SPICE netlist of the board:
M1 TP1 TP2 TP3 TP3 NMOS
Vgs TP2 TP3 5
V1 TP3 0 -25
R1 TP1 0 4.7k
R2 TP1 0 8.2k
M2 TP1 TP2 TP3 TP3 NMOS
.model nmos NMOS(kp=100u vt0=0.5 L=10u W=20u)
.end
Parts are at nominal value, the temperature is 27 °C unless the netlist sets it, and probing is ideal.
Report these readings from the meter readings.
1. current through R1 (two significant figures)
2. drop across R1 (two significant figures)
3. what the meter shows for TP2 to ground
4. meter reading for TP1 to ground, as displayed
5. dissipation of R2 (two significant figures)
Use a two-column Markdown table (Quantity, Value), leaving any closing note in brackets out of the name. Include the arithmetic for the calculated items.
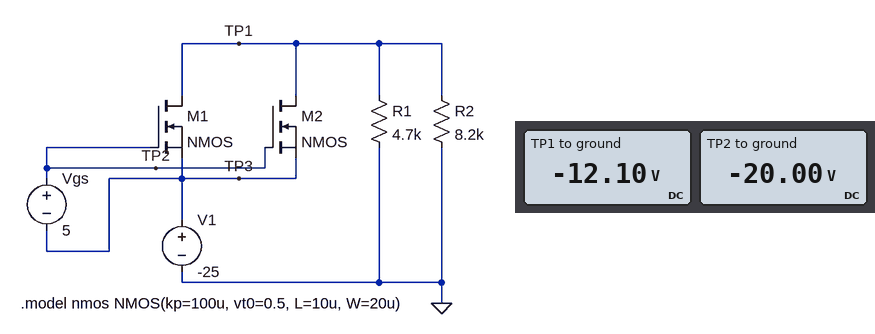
| Quantity | Value |
|---|---|
| current through R1 | (0 V - (-12.1 V)) / 4.7 kΩ = 2.6 mA |
| drop across R1 | 0 V - (-12.1 V) = 12 V |
| what the meter shows for TP2 to ground | -20.00 V |
| meter reading for TP1 to ground, as displayed | -12.10 V |
| dissipation of R2 | (0 V - (-12.1 V))^2 / 8.2 kΩ = 18 mW |
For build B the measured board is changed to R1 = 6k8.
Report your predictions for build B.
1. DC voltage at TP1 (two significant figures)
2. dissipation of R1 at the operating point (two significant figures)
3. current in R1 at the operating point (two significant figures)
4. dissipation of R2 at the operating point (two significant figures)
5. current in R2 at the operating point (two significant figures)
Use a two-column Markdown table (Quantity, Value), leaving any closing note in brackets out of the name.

| Quantity | Value |
|---|---|
| DC voltage at TP1 | -15 V |
| dissipation of R1 at the operating point | 33 mW |
| current in R1 at the operating point | 2.2 mA |
| dissipation of R2 at the operating point | 28 mW |
| current in R2 at the operating point | 1.8 mA |
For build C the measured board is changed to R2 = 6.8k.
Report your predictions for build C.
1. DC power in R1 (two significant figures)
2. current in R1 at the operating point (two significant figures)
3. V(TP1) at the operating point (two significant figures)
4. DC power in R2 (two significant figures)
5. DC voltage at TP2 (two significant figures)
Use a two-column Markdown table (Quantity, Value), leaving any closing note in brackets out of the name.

| Quantity | Value |
|---|---|
| DC power in R1 | 27 mW |
| current in R1 at the operating point | 2.4 mA |
| V(TP1) at the operating point | -11 V |
| DC power in R2 | 19 mW |
| DC voltage at TP2 | -20 V |
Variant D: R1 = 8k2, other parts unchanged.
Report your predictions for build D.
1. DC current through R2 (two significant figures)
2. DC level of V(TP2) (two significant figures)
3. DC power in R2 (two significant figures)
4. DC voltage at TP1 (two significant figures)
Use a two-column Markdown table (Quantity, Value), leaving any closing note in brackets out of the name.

| Quantity | Value |
|---|---|
| DC current through R2 | 2.0 mA |
| DC level of V(TP2) | -20 V |
| DC power in R2 | 34 mW |
| DC voltage at TP1 | -17 V |
